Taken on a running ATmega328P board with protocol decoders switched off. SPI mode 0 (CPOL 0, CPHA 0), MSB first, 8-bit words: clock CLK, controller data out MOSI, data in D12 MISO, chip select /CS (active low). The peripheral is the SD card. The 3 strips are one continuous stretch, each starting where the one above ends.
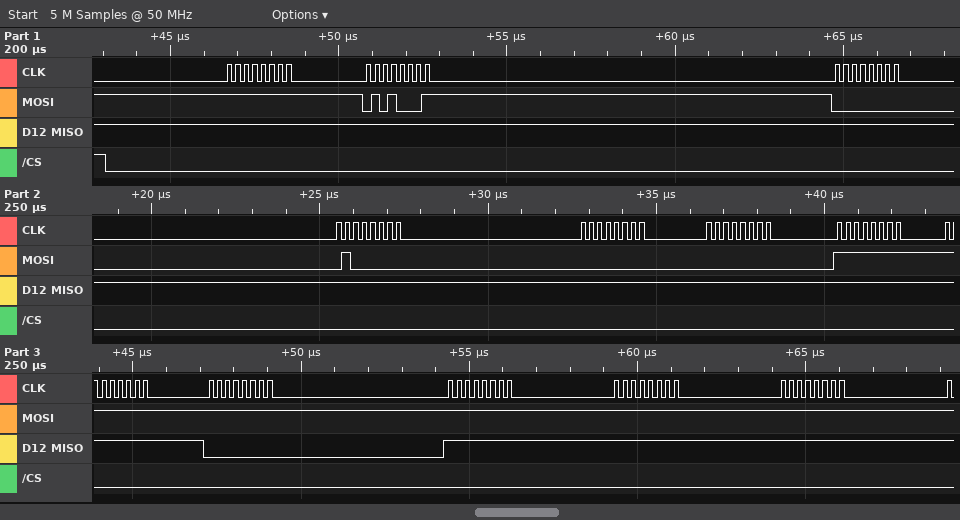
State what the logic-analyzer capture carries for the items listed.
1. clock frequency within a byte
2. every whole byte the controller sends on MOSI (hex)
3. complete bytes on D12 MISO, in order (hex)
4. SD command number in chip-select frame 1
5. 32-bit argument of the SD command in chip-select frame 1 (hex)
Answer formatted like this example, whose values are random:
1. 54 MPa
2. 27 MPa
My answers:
1. 4 MHz
2. 0xFF 0x51 0x00 0x40 0x00 0x00 0xFF 0xFF 0xFF 0xFF 0xFF 0xFF
3. 0xFF 0xFF 0xFF 0xFF 0xFF 0xFF 0xFF 0xFF 0x00 0xFF 0xFF 0xFF
4. CMD17
5. 0x00400000
